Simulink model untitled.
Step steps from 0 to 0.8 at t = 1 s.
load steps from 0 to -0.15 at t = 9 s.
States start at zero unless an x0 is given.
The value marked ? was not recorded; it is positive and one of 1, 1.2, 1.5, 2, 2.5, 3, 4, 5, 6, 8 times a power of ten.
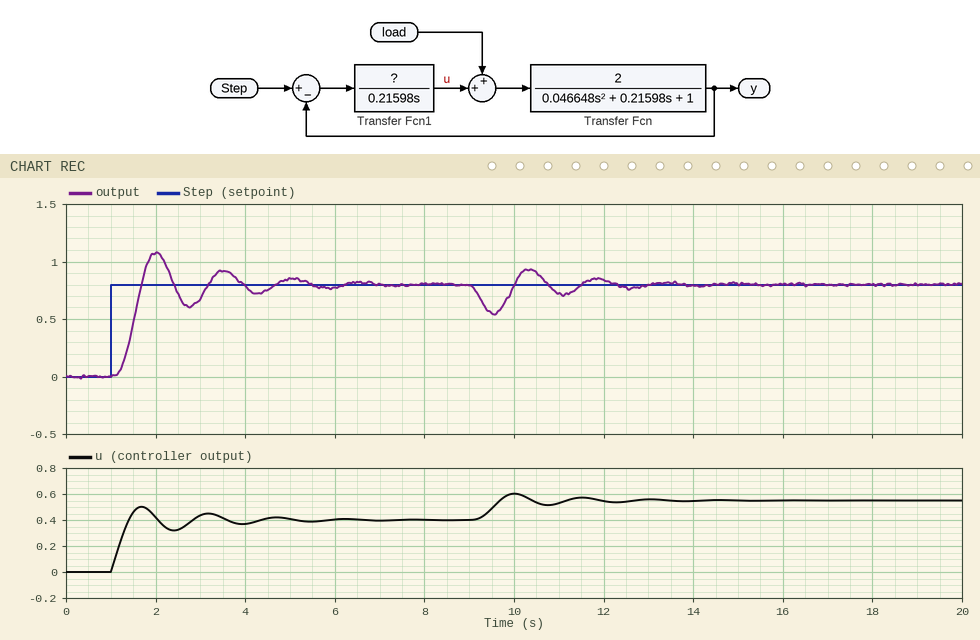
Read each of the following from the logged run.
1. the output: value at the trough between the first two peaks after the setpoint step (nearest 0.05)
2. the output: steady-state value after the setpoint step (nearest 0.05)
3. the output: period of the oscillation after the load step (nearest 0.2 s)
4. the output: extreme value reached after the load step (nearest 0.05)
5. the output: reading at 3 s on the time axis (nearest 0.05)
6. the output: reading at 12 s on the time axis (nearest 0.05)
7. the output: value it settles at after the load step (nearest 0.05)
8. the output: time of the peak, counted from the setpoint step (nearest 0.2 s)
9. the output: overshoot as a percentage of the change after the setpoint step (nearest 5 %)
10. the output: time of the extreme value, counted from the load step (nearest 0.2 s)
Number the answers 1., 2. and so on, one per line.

1. 0.60
2. 0.80
3. 1.6 s
4. 0.55
5. 0.70
6. 0.85
7. 0.80
8. 1.0 s
9. 35 %
10. 0.6 s
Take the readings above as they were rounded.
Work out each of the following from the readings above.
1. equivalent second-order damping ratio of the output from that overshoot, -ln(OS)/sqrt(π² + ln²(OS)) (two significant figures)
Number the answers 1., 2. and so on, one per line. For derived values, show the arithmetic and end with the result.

1. ln(0.35) = -1.050; 1.050 / sqrt(9.870 + 1.102) = 0.32
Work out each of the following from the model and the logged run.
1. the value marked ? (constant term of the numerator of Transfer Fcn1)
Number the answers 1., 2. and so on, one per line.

1. 0.3
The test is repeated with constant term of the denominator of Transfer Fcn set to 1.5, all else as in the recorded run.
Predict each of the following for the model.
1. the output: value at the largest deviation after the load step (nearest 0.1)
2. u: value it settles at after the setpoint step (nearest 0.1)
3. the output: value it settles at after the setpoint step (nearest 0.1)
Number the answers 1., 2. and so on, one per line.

1. 0.6
2. 0.6
3. 0.8
